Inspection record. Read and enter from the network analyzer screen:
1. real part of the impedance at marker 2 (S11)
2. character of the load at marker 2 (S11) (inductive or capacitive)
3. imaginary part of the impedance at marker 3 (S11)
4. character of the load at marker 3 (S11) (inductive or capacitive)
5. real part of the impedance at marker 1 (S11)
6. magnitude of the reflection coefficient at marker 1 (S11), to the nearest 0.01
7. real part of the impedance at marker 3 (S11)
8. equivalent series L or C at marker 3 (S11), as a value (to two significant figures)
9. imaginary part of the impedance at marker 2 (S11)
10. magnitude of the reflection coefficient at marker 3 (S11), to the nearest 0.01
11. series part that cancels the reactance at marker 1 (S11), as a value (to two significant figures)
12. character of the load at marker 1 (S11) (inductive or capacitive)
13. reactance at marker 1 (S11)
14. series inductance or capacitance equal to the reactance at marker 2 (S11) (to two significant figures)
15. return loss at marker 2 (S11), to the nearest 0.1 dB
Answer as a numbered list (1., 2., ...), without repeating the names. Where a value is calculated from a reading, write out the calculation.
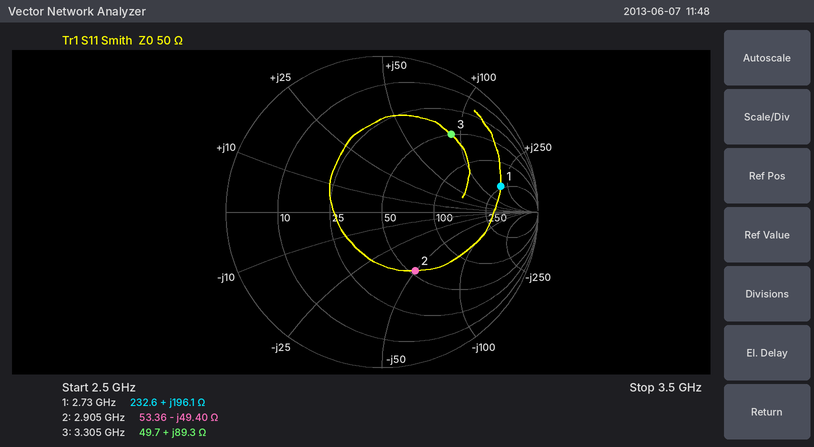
1. 53.36 Ω
2. capacitive
3. +89.3 Ω
4. inductive
5. 232.6 Ω
6. 0.78
7. 49.7 Ω
8. L = 89.3 Ω/(2π × 3.305 GHz) ≈ 4.3 nH
9. -49.40 Ω
10. 0.67
11. C = 1/(2π × 2.73 GHz × 196.1 Ω) ≈ 297 fF, so 300 fF to two significant figures
12. inductive
13. +196.1 Ω
14. C = 1/(2π × 2.905 GHz × 49.4 Ω) ≈ 1.1 pF
15. 7.3 dB
